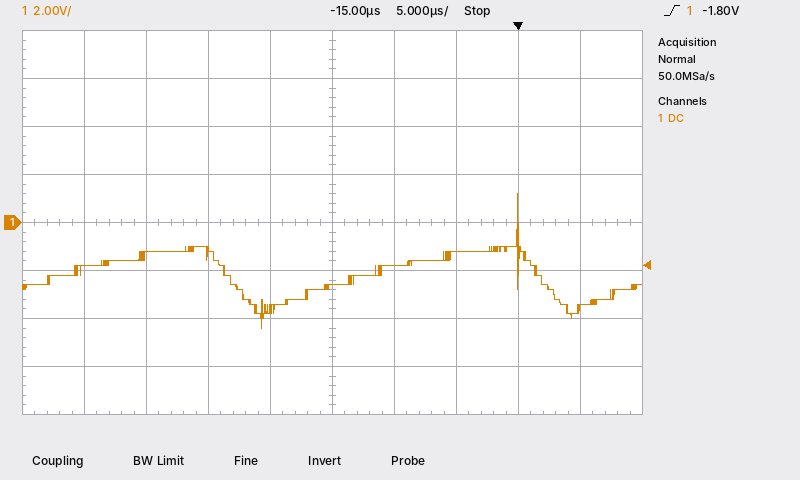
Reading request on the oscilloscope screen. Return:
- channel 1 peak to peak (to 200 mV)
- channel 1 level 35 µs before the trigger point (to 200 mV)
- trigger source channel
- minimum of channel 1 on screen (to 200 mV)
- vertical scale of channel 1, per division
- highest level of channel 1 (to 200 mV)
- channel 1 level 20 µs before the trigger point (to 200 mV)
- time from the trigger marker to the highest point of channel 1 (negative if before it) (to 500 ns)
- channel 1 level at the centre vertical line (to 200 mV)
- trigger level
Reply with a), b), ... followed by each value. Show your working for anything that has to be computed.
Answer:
a) 1.2 V − (-4.4 V) = 5.6 V
b) -1.8 V
c) channel 1
d) -4.4 V
e) 2 V
f) 1.2 V
g) -3.6 V
h) 0.0 µs
i) -2.6 V
j) -1.80 V
